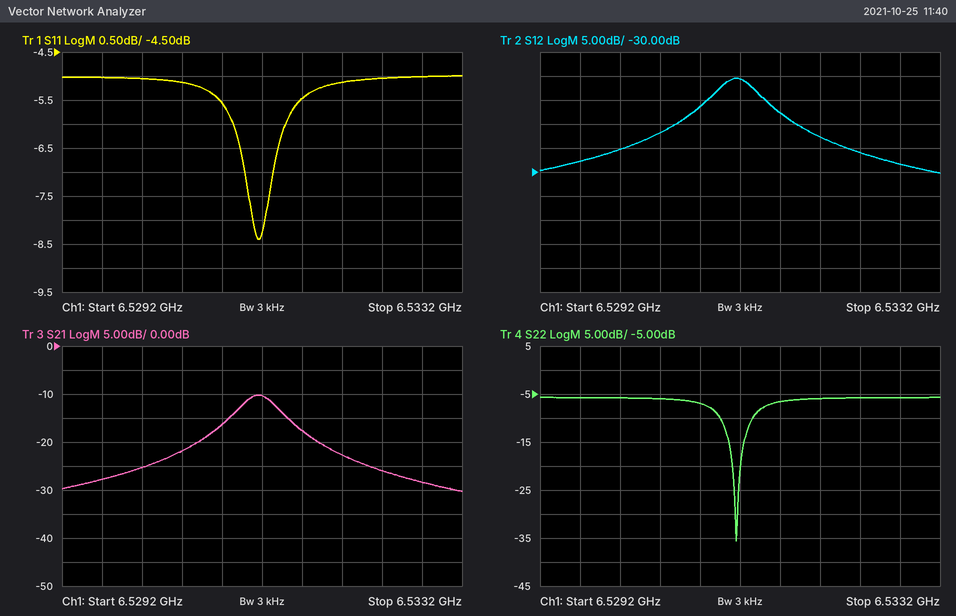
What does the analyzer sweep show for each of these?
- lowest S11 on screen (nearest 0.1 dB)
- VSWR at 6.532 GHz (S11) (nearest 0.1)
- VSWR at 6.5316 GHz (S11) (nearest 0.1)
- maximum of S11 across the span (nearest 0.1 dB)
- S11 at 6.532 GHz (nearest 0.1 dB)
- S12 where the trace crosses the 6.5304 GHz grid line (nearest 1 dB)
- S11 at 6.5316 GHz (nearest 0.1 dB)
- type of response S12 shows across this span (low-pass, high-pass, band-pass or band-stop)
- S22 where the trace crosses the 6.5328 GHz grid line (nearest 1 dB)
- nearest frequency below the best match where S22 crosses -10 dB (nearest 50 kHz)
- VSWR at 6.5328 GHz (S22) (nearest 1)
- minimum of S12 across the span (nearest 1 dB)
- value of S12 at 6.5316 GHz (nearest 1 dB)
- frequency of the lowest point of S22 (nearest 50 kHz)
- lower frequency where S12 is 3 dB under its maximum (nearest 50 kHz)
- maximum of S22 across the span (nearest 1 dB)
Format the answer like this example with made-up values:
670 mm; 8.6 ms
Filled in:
-8.4 dB; 3.5; 3.3; -5.0 dB; -5.1 dB; -22 dB; -5.5 dB; band-pass; -6 dB; 6.53100 GHz; 3; -30 dB; -18 dB; 6.53115 GHz; 6.53095 GHz; -6 dB
